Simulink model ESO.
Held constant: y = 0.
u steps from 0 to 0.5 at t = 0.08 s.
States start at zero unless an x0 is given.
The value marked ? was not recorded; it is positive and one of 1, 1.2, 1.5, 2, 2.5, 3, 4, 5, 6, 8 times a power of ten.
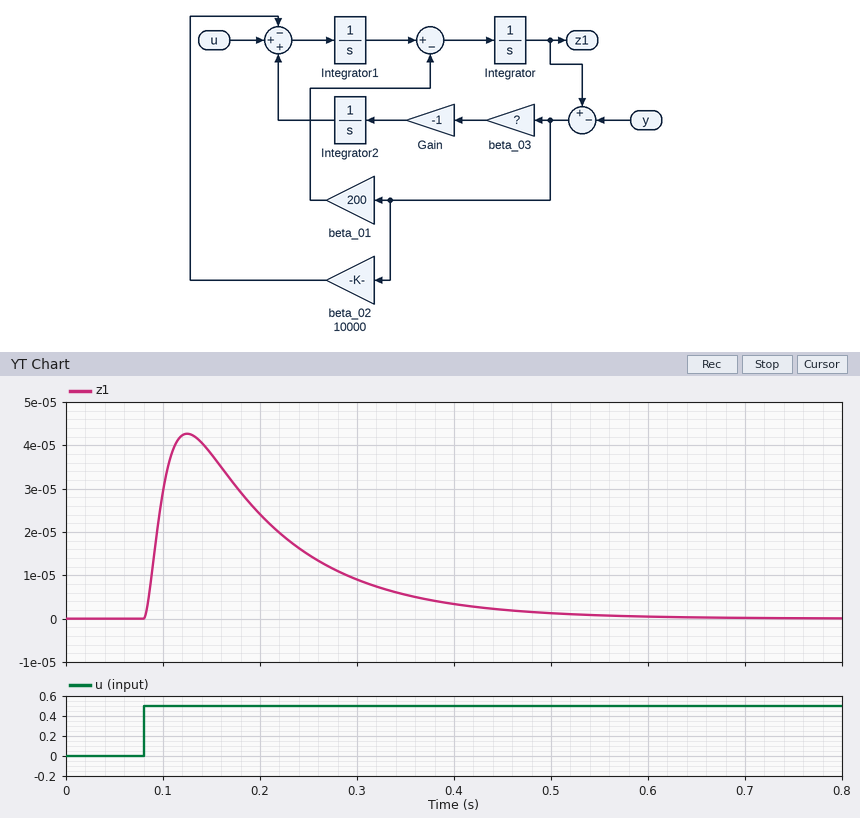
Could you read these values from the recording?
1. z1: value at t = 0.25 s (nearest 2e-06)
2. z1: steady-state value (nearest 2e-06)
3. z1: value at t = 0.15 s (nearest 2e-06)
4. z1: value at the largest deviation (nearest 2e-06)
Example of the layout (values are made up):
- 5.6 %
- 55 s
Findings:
- 0.000014
- 0.000000
- 0.000038
- 0.000042
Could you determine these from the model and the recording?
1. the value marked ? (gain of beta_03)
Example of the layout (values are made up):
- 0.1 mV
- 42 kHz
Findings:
- 80000
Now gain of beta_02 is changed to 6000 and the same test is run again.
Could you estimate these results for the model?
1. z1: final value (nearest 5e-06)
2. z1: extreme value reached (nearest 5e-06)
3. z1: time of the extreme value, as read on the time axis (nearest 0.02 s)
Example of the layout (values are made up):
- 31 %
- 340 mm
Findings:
- 0.000000
- 0.000060
- 0.14 s
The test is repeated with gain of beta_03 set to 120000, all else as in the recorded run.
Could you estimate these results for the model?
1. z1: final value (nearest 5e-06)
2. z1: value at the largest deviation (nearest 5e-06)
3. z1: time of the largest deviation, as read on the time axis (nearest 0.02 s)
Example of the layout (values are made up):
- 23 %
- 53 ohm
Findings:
- 0.000000
- 0.000040
- 0.12 s
